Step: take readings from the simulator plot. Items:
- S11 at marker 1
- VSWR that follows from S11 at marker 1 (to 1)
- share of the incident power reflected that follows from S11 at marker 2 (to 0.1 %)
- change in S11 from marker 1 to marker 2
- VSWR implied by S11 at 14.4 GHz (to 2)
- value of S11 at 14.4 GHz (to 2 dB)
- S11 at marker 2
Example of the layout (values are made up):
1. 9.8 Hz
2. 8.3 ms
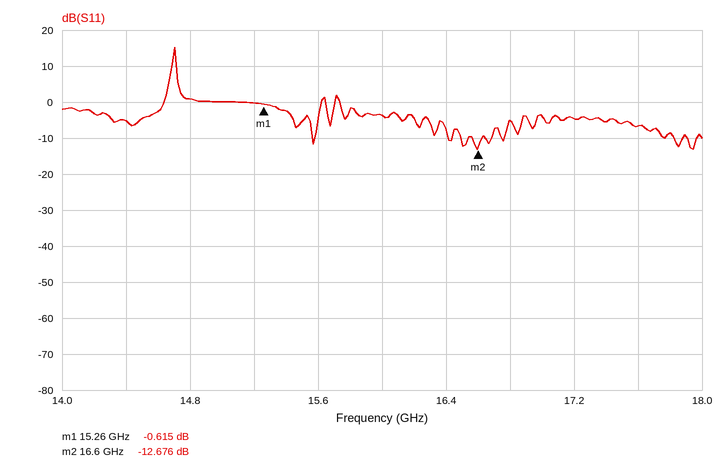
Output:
1. -0.615 dB
2. 28
3. 5.4 %
4. -12.061 dB
5. 4
6. -6 dB
7. -12.676 dB
